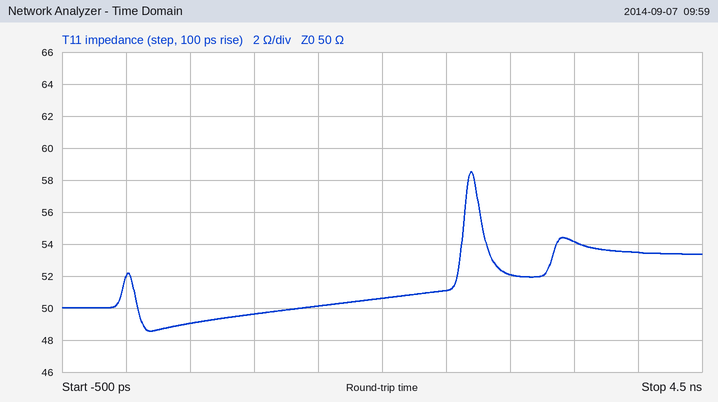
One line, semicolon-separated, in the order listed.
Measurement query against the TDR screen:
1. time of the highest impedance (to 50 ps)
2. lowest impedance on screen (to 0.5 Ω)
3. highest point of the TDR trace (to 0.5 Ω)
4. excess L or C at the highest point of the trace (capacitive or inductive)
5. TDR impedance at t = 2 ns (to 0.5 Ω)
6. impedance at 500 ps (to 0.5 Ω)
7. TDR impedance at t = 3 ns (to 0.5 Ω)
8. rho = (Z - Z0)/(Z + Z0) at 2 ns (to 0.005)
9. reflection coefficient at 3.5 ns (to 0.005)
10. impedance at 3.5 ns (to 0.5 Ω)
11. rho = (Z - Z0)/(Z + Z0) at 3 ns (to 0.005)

2.70 ns; 48.5 Ω; 58.5 Ω; inductive; 50.5 Ω; 49.0 Ω; 52.0 Ω; +0.005; +0.040; 54.0 Ω; +0.020
